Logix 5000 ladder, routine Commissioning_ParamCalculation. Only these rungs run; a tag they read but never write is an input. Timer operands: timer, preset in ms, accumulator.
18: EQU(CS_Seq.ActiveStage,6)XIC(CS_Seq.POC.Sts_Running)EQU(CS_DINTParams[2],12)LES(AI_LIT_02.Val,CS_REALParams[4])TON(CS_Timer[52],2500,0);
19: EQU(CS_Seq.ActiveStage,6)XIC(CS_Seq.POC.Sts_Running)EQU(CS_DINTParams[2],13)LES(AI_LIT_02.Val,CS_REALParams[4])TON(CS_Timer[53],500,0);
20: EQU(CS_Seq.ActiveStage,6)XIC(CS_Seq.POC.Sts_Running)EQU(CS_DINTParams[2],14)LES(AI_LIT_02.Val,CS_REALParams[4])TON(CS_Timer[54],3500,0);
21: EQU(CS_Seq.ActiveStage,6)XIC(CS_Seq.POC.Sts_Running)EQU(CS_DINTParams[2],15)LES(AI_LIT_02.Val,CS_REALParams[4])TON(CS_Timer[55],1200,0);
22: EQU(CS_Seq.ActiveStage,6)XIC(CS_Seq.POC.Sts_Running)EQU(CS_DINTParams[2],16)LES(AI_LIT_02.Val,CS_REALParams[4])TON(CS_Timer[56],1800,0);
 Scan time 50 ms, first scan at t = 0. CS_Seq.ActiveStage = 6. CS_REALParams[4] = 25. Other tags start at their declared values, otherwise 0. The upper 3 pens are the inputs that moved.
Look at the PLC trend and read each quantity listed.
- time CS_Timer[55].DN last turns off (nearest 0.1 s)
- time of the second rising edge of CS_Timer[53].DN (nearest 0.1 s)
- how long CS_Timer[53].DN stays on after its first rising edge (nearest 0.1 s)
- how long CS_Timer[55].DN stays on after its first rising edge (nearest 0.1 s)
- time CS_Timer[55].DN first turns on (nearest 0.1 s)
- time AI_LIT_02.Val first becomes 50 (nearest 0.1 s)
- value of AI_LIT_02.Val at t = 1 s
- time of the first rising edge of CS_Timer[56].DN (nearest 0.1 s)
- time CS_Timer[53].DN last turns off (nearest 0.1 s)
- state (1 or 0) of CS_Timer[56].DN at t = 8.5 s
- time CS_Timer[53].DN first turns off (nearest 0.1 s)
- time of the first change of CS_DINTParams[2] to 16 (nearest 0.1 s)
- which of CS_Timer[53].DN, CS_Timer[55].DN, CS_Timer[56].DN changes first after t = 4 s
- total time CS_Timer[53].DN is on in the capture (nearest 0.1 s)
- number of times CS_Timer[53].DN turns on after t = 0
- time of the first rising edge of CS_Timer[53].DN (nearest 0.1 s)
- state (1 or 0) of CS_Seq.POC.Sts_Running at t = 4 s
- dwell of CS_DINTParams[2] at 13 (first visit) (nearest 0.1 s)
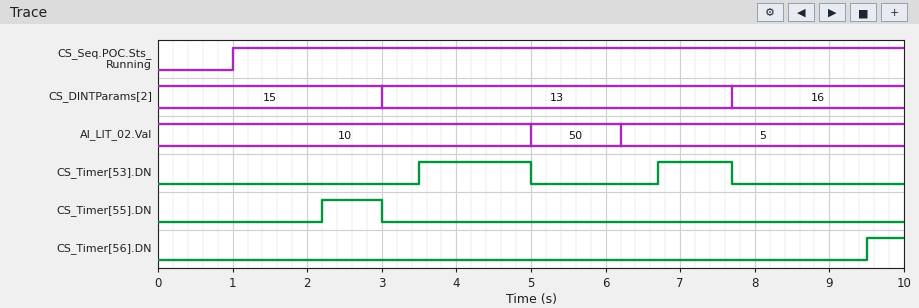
3.0 s
6.7 s
1.5 s
0.8 s
2.2 s
5.0 s
10
9.5 s
7.7 s
0
5.0 s
7.7 s
CS_Timer[53].DN
2.5 s
2
3.5 s
1
4.7 s
